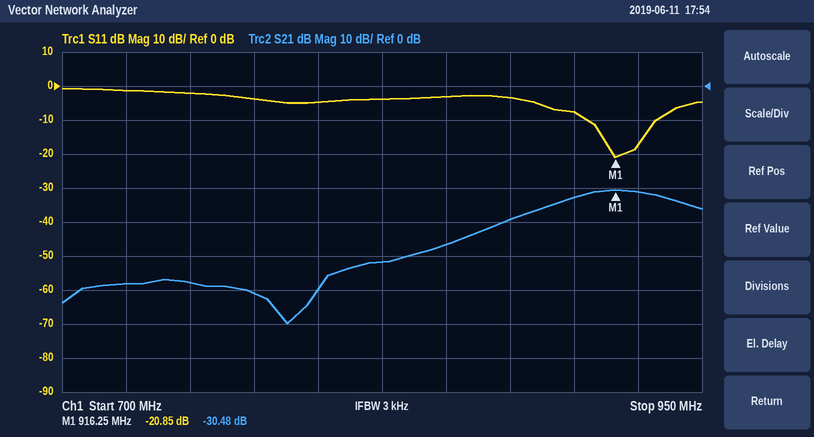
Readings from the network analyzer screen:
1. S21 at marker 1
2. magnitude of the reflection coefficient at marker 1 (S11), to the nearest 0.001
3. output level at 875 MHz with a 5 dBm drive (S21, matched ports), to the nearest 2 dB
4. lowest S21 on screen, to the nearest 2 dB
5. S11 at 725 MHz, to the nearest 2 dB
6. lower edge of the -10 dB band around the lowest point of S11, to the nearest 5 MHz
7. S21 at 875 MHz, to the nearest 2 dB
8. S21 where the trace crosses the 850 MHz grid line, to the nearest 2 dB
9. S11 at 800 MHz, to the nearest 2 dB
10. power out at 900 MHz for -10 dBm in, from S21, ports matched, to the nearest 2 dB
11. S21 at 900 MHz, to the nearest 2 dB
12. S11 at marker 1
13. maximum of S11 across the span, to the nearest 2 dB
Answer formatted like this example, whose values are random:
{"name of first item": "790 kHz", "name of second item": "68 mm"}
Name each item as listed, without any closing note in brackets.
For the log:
{"S21 at marker 1": "-30.48 dB", "magnitude of the reflection coefficient at marker 1 (S11), to the nearest 0.001": "0.091", "output level at 875 MHz with a 5 dBm drive (S21, matched ports), to the nearest 2 dB": "-34 dBm", "lowest S21 on screen, to the nearest 2 dB": "-70 dB", "S11 at 725 MHz, to the nearest 2 dB": "-2 dB", "lower edge of the -10 dB band around the lowest point of S11, to the nearest 5 MHz": "905 MHz", "S21 at 875 MHz, to the nearest 2 dB": "-40 dB", "S21 where the trace crosses the 850 MHz grid line, to the nearest 2 dB": "-46 dB", "S11 at 800 MHz, to the nearest 2 dB": "-4 dB", "power out at 900 MHz for -10 dBm in, from S21, ports matched, to the nearest 2 dB": "-42 dBm", "S21 at 900 MHz, to the nearest 2 dB": "-32 dB", "S11 at marker 1": "-20.85 dB", "maximum of S11 across the span, to the nearest 2 dB": "0 dB"}
